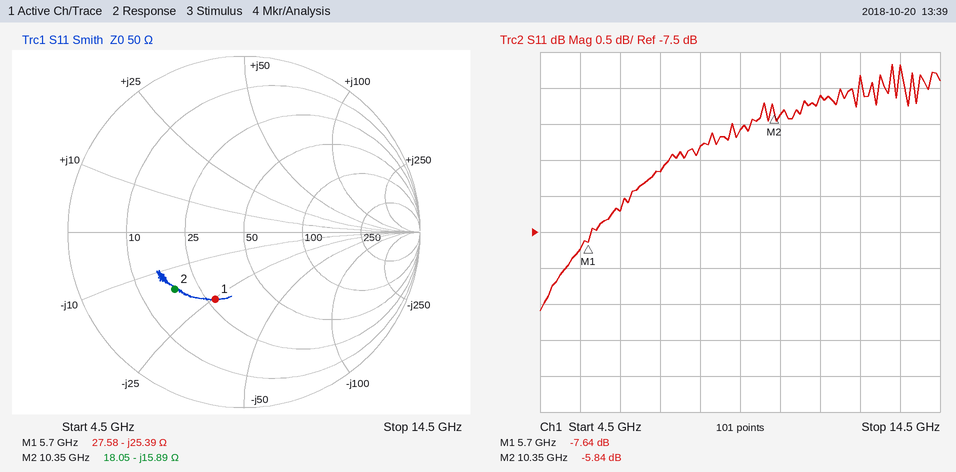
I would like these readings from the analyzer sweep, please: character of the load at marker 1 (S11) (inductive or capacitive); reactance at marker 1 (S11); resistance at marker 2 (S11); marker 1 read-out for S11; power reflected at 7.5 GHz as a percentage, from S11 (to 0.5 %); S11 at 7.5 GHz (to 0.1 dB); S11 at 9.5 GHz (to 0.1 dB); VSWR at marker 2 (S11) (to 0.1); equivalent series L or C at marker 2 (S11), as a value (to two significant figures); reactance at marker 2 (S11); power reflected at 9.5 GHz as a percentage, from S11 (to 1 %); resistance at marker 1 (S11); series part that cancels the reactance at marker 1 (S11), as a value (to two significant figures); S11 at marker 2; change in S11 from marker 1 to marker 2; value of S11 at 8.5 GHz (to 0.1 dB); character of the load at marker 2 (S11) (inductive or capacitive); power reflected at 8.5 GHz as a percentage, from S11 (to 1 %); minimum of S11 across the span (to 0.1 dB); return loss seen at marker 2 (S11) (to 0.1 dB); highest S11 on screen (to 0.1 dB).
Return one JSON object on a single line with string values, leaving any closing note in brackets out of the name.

{"character of the load at marker 1 (S11)": "capacitive", "reactance at marker 1": "-25.39 Ω", "resistance at marker 2": "18.05 Ω", "marker 1 read-out for S11": "-7.64 dB", "power reflected at 7.5 GHz as a percentage, from S11": "21.5 %", "S11 at 7.5 GHz": "-6.7 dB", "S11 at 9.5 GHz": "-6.1 dB", "VSWR at marker 2 (S11)": "3.1", "equivalent series L or C at marker 2 (S11), as a value": "970 fF", "reactance at marker 2": "-15.89 Ω", "power reflected at 9.5 GHz as a percentage, from S11": "25 %", "resistance at marker 1": "27.58 Ω", "series part that cancels the reactance at marker 1 (S11), as a value": "710 pH", "S11 at marker 2": "-5.84 dB", "change in S11 from marker 1 to marker 2": "1.80 dB", "value of S11 at 8.5 GHz": "-6.3 dB", "character of the load at marker 2 (S11)": "capacitive", "power reflected at 8.5 GHz as a percentage, from S11": "23 %", "minimum of S11 across the span": "-8.6 dB", "return loss seen at marker 2 (S11)": "5.8 dB", "highest S11 on screen": "-5.2 dB"}
